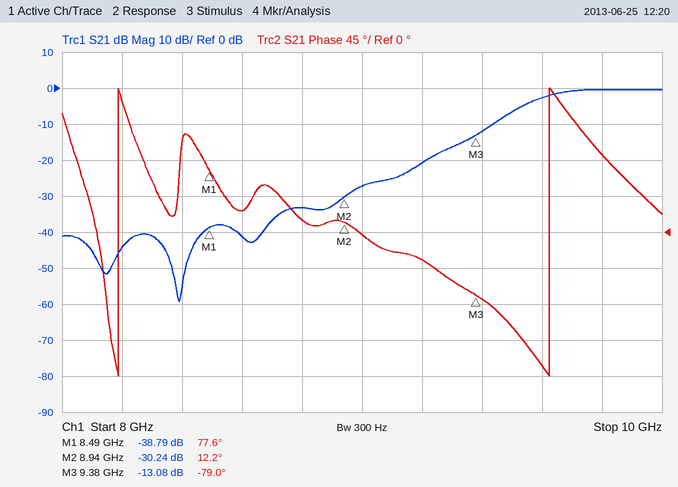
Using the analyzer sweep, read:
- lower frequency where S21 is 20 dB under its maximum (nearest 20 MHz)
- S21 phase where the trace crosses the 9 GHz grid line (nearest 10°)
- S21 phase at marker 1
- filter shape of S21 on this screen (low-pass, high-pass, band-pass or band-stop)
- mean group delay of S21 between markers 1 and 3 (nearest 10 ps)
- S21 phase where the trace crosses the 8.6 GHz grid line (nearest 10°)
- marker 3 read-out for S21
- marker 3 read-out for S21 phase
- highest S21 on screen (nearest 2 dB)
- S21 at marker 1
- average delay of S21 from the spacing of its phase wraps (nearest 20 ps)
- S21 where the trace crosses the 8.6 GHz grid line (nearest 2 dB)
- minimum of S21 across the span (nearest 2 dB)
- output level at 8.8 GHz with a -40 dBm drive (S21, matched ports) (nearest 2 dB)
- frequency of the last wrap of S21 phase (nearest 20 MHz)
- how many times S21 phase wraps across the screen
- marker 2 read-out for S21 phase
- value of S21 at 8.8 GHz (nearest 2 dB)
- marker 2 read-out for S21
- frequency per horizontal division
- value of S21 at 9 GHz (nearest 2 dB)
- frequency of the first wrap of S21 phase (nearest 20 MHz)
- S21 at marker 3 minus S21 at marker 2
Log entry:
9.20 GHz
0°
77.6°
high-pass
490 ps
30°
-13.08 dB
-79.0°
0 dB
-38.79 dB
700 ps
-42 dB
-60 dB
-74 dBm
9.62 GHz
2
12.2°
-34 dB
-30.24 dB
200 MHz
-28 dB
8.18 GHz
17.16 dB
